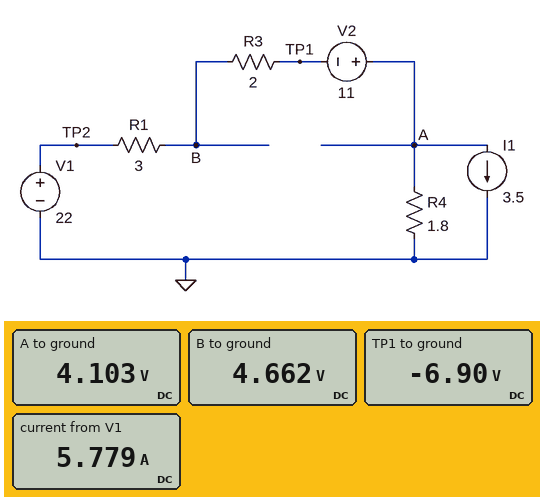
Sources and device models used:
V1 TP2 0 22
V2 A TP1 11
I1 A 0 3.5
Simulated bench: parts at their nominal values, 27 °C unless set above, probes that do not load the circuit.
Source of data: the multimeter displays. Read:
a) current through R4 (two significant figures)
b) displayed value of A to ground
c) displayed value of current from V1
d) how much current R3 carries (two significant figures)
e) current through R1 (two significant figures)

2.3 A
4.103 V
5.779 A
5.8 A
5.8 A
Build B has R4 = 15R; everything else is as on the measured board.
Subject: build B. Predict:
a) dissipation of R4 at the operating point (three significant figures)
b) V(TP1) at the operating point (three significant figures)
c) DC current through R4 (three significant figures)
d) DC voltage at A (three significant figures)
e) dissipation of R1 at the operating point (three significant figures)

9.01 W
625 mV
775 mA
11.6 V
54.8 W
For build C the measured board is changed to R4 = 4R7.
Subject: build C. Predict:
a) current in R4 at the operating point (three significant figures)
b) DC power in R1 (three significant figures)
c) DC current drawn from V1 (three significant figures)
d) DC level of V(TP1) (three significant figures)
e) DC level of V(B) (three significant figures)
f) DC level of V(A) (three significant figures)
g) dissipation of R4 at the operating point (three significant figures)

1.60 A
78.0 W
5.10 A
-3.49 V
6.71 V
7.51 V
12.0 W
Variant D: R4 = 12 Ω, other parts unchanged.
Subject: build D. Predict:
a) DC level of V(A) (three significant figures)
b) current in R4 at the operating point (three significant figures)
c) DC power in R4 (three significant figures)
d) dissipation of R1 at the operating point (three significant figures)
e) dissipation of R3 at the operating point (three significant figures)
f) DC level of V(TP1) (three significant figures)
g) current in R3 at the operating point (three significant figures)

10.9 V
912 mA
9.98 W
58.4 W
38.9 W
-58.8 mV
4.41 A
